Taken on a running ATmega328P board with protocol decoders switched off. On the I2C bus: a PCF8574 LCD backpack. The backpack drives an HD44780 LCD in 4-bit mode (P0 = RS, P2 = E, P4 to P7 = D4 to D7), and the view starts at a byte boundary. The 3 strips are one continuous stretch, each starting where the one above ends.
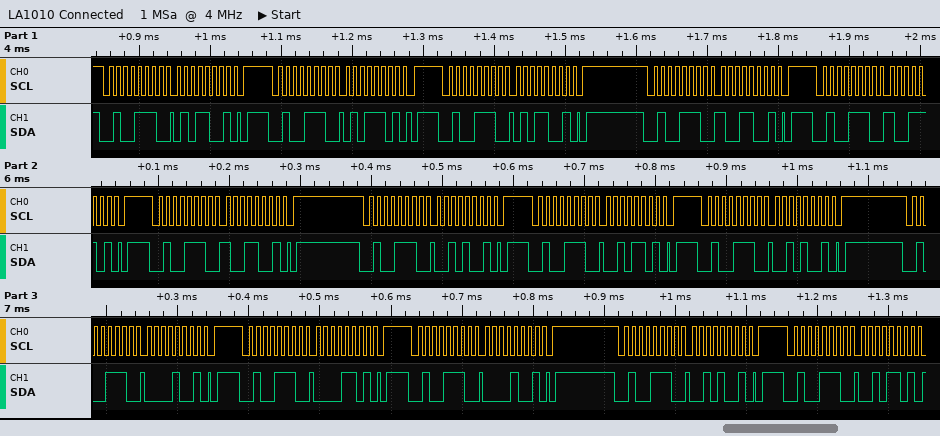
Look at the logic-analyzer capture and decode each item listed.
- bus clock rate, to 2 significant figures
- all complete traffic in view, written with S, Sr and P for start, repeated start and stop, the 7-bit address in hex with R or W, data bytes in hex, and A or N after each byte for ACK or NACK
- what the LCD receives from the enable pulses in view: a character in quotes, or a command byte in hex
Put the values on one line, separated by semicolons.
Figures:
100 kHz; S 27W A 59 A P S 27W A 5D A P S 27W A 59 A P S 27W A 99 A P S 27W A 9D A P S 27W A 99 A P S 27W A 29 A P S 27W A 2D A P S 27W A 29 A P S 27W A 09 A P S 27W A 0D A P S 27W A 09 A P S 27W A 29 A P S 27W A 2D A; 'Y' ' '
